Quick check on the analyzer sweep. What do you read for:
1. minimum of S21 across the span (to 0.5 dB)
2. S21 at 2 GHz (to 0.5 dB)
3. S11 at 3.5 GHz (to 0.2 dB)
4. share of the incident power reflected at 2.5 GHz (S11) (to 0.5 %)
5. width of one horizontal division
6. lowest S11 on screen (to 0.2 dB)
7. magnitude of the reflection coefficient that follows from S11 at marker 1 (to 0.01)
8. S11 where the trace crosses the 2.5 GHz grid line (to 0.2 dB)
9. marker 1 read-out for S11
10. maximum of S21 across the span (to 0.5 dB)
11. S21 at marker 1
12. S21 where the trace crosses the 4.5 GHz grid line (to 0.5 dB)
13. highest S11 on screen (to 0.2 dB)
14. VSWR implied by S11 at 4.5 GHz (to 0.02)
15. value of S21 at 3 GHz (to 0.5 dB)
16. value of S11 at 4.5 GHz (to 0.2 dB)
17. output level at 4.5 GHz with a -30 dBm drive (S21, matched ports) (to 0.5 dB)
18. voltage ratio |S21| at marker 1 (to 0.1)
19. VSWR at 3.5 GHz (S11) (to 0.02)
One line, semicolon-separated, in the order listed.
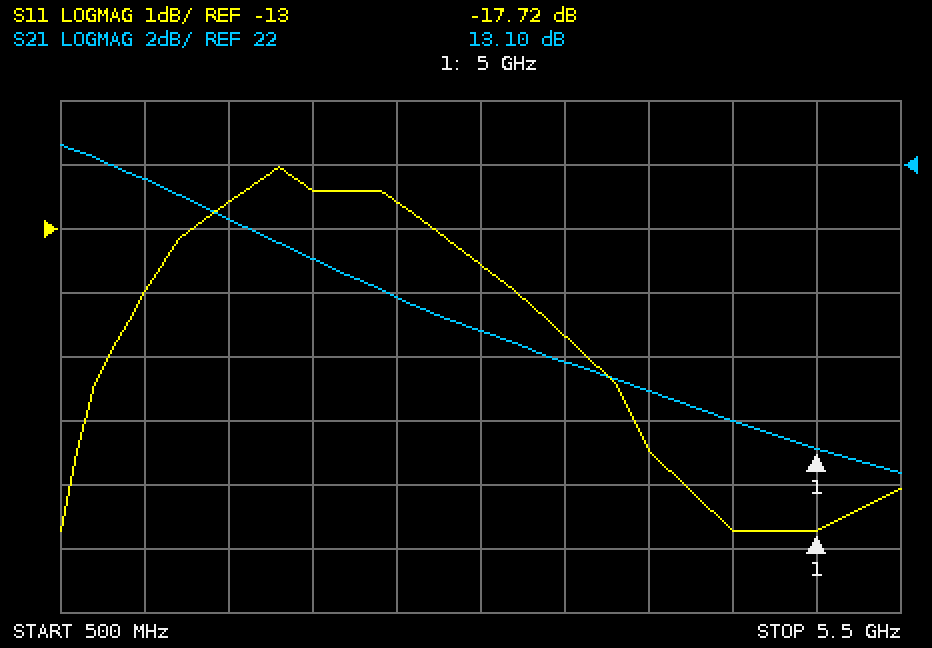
12.5 dB; 19.0 dB; -14.6 dB; 5.5 %; 500 MHz; -17.8 dB; 0.13; -12.6 dB; -17.72 dB; 22.5 dB; 13.10 dB; 14.0 dB; -12.0 dB; 1.30; 17.0 dB; -17.8 dB; -16.0 dBm; 4.5; 1.46
